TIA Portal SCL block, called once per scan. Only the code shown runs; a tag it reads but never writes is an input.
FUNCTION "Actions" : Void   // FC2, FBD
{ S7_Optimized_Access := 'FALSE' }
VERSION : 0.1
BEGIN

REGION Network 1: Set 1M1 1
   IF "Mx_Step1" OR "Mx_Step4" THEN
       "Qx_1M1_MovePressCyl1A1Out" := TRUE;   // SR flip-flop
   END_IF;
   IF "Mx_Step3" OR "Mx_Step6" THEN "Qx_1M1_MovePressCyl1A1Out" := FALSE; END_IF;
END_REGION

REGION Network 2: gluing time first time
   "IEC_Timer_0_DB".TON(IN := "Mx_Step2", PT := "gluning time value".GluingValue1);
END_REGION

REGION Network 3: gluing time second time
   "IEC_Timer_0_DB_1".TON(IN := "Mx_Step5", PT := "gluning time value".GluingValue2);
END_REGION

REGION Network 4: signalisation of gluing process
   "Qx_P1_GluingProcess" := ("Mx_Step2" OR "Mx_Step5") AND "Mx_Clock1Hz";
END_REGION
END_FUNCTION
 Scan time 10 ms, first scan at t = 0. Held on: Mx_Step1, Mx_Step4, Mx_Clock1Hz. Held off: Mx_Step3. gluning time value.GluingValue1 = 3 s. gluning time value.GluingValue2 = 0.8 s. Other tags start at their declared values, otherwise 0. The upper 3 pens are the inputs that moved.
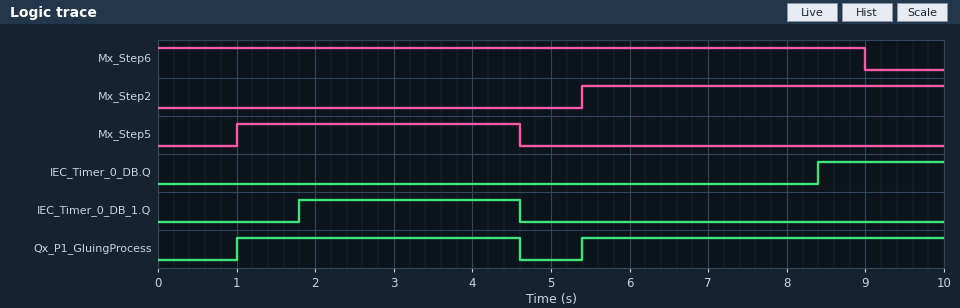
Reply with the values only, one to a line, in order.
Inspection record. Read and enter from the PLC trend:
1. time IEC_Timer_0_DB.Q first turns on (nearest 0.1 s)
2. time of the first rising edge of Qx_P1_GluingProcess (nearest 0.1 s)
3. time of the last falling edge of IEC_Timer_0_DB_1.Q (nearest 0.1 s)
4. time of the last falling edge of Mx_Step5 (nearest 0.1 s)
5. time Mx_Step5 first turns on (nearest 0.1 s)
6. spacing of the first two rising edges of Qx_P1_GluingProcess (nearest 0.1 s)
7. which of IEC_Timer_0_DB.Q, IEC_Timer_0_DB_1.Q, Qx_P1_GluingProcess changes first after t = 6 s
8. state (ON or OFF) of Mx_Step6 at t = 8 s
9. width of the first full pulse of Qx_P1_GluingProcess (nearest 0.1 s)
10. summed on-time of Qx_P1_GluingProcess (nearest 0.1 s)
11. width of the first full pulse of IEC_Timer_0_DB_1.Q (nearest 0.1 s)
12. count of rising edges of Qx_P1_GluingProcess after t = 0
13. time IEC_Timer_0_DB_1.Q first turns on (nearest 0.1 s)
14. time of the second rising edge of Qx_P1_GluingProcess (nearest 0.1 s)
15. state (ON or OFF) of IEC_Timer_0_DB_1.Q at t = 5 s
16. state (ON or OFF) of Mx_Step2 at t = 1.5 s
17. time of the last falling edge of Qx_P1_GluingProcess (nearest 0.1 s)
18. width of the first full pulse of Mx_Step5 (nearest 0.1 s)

8.4 s
1.0 s
4.6 s
4.6 s
1.0 s
4.4 s
IEC_Timer_0_DB.Q
ON
3.6 s
8.2 s
2.8 s
2
1.8 s
5.4 s
OFF
OFF
4.6 s
3.6 s
